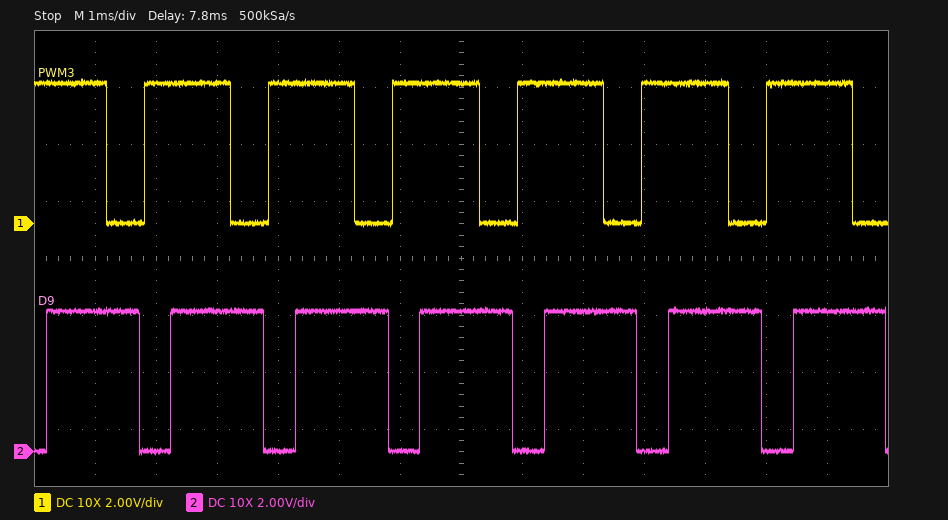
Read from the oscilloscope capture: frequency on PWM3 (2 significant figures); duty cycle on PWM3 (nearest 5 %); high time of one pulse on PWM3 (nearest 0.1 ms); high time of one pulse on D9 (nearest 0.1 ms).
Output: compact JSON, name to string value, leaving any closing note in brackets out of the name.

{"frequency on PWM3": "490 Hz", "duty cycle on PWM3": "70 %", "high time of one pulse on PWM3": "1.4 ms", "high time of one pulse on D9": "1.5 ms"}
